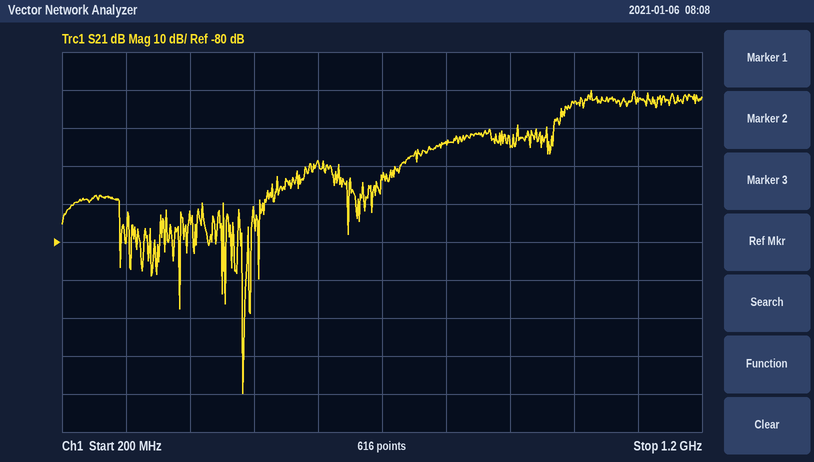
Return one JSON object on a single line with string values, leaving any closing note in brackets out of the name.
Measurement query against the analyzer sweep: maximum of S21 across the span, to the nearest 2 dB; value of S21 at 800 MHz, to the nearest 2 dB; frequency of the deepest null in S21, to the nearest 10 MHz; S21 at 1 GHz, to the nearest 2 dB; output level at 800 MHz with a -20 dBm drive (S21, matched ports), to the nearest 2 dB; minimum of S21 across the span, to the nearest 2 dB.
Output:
{"maximum of S21 across the span, to the nearest 2 dB": "-40 dB", "value of S21 at 800 MHz, to the nearest 2 dB": "-54 dB", "frequency of the deepest null in S21, to the nearest 10 MHz": "480 MHz", "S21 at 1 GHz, to the nearest 2 dB": "-44 dB", "output level at 800 MHz with a -20 dBm drive (S21, matched ports), to the nearest 2 dB": "-74 dBm", "minimum of S21 across the span, to the nearest 2 dB": "-120 dB"}
